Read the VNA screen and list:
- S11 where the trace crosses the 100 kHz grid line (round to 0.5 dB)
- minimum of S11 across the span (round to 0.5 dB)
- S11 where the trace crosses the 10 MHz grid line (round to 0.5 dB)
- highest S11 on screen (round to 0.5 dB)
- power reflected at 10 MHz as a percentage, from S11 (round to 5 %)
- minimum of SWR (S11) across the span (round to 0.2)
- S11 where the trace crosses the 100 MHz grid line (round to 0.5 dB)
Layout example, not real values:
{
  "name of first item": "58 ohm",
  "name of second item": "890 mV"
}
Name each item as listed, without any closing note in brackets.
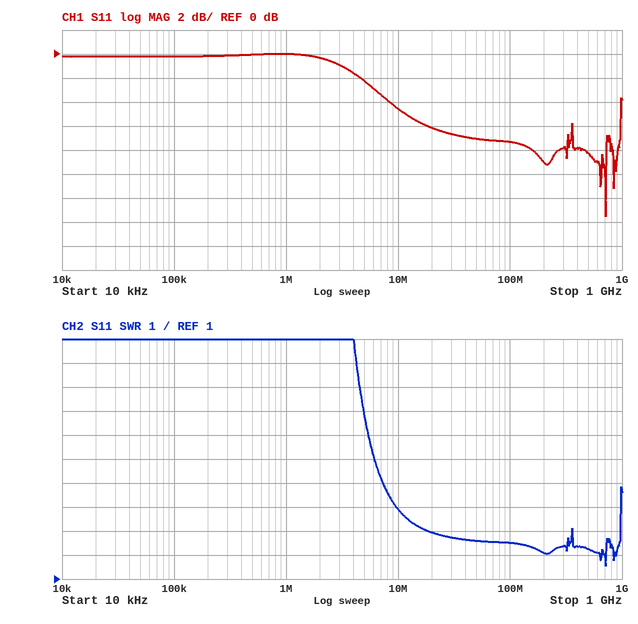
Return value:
{
  "S11 where the trace crosses the 100 kHz grid line": "0.0 dB",
  "minimum of S11 across the span": "-13.5 dB",
  "S11 where the trace crosses the 10 MHz grid line": "-4.5 dB",
  "highest S11 on screen": "0.0 dB",
  "power reflected at 10 MHz as a percentage, from S11": "35 %",
  "minimum of SWR (S11) across the span": "1.6",
  "S11 where the trace crosses the 100 MHz grid line": "-7.5 dB"
}
